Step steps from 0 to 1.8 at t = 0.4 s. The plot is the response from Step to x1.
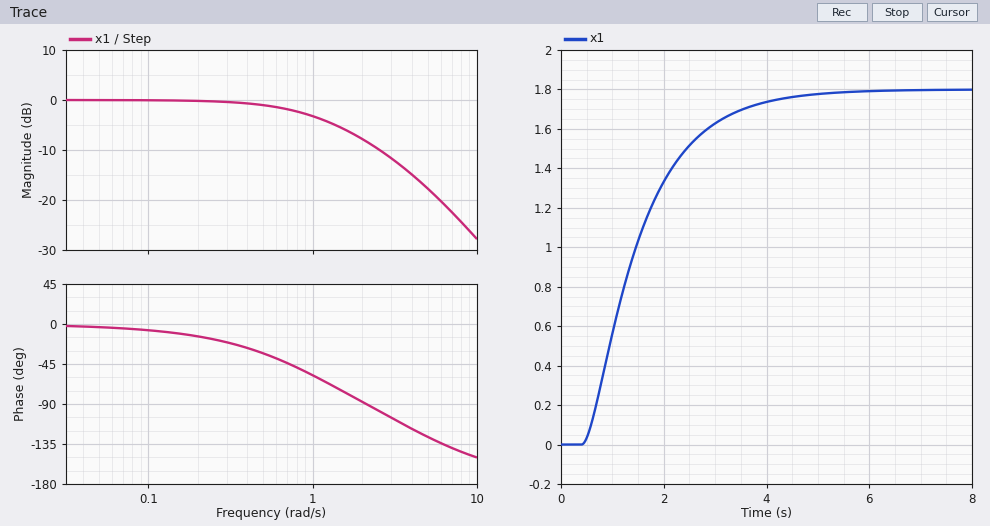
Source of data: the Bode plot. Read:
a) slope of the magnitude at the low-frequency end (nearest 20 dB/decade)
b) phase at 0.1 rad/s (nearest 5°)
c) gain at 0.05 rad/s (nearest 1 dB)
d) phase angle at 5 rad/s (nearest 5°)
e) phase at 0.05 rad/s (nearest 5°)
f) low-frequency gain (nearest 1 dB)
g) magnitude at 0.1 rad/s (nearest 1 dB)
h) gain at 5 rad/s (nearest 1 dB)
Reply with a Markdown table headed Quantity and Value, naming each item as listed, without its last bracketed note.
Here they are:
| Quantity | Value |
|---|---|
| slope of the magnitude at the low-frequency end | 0 dB/decade |
| phase at 0.1 rad/s | -5° |
| gain at 0.05 rad/s | 0 dB |
| phase angle at 5 rad/s | -125° |
| phase at 0.05 rad/s | -5° |
| low-frequency gain | 0 dB |
| magnitude at 0.1 rad/s | 0 dB |
| gain at 5 rad/s | -18 dB |
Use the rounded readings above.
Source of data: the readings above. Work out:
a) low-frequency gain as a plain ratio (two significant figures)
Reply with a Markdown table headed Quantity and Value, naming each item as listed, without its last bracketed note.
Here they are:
| Quantity | Value |
|---|---|
| low-frequency gain as a plain ratio | 1.0 |
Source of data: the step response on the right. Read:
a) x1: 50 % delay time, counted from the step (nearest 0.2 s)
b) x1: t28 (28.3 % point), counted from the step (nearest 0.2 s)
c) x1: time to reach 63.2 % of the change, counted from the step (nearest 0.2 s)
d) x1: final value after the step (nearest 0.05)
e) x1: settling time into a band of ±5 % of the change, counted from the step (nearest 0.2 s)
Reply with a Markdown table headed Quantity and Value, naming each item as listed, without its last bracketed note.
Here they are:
| Quantity | Value |
|---|---|
| x1: 50 % delay time, counted from the step | 1.0 s |
| x1: t28 (28.3 % point), counted from the step | 0.6 s |
| x1: time to reach 63.2 % of the change, counted from the step | 1.2 s |
| x1: final value after the step | 1.80 |
| x1: settling time into a band of ±5 % of the change, counted from the step | 3.2 s |
